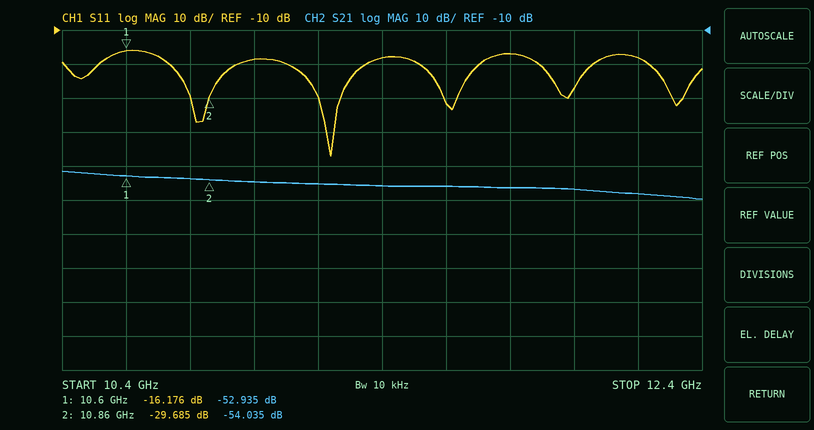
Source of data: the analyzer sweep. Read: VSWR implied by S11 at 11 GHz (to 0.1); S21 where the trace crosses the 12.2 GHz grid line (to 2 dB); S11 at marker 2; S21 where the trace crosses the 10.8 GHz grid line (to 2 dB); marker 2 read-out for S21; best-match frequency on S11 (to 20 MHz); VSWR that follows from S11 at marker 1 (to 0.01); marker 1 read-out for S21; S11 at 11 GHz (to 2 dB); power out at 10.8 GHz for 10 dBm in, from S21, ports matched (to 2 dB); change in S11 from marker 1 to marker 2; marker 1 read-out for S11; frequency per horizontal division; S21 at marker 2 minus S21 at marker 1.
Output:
1.3
-58 dB
-29.685 dB
-54 dB
-54.035 dB
11.24 GHz
1.37
-52.935 dB
-18 dB
-44 dBm
-13.509 dB
-16.176 dB
200 MHz
-1.100 dB
